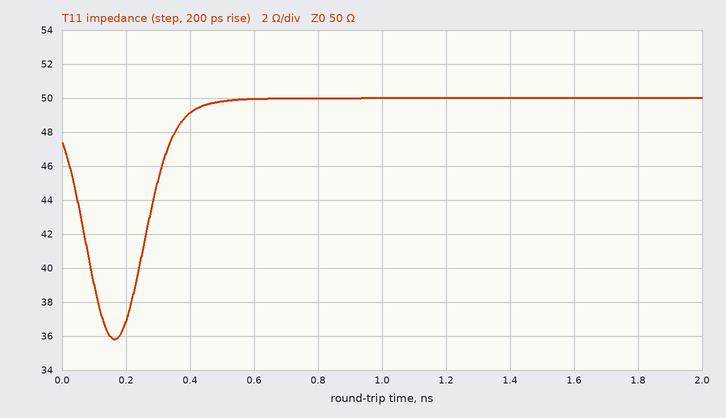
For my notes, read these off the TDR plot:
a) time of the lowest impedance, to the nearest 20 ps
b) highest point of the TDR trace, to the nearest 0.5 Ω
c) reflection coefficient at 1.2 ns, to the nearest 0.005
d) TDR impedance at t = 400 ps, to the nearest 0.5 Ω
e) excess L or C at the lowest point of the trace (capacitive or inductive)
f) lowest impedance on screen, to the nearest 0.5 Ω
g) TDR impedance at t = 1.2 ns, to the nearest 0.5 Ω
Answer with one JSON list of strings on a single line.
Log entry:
["160 ps", "50.0 Ω", "0.000", "49.0 Ω", "capacitive", "36.0 Ω", "50.0 Ω"]
